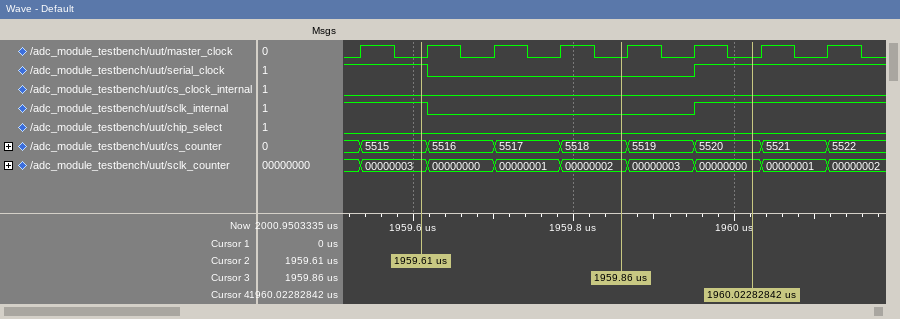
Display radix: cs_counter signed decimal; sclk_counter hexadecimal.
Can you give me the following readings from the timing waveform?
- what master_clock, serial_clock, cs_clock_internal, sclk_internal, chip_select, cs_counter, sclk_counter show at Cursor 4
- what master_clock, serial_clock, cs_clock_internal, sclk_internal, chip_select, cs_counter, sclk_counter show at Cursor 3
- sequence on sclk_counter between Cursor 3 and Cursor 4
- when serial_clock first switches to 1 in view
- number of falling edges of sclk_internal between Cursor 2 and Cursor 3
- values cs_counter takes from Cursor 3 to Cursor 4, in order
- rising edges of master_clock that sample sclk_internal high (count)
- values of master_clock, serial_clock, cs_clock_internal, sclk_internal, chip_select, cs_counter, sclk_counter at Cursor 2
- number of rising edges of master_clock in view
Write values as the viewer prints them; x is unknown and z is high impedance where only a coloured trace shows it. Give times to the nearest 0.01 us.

master_clock=0, serial_clock=1, cs_clock_internal=0, sclk_internal=1, chip_select=0, cs_counter=5520, sclk_counter=00000000
master_clock=0, serial_clock=0, cs_clock_internal=0, sclk_internal=0, chip_select=0, cs_counter=5518, sclk_counter=00000002
00000002, 00000003, 00000000
1959.95 us
1
5518, 5519, 5520
4
master_clock=0, serial_clock=1, cs_clock_internal=0, sclk_internal=1, chip_select=0, cs_counter=5515, sclk_counter=00000003
8
